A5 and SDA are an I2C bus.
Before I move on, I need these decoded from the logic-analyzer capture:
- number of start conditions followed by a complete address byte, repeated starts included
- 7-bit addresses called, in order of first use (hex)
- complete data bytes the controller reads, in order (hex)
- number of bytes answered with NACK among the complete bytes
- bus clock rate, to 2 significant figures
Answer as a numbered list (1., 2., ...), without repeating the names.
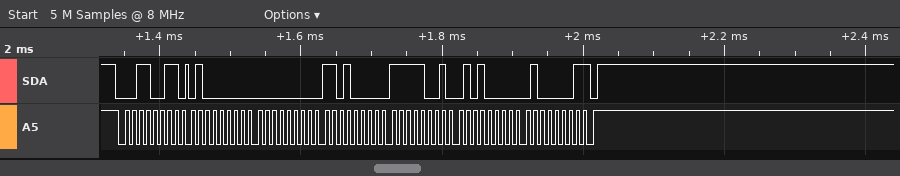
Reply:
1. 1
2. 0x19
3. 40 00 D0 F9 50 41
4. 1
5. 100 kHz
